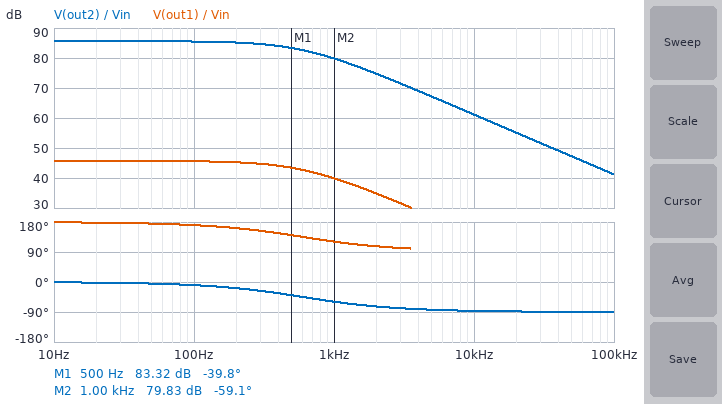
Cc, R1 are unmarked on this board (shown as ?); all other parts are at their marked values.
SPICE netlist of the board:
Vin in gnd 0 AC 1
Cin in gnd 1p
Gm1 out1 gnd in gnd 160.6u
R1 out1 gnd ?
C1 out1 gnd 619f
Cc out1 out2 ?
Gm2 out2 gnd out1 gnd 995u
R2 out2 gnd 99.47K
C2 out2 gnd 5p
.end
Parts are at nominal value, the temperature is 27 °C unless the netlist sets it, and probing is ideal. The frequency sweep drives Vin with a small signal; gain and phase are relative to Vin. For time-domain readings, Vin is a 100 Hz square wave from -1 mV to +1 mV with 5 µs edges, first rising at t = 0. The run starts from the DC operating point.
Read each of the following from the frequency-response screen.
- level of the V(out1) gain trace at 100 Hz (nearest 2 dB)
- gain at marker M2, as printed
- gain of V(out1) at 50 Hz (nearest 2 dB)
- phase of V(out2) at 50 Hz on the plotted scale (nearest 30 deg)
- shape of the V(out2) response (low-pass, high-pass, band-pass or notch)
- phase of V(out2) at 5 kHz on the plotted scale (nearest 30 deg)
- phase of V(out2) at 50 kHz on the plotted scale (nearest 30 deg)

46 dB
79.83 dB
46 dB
0 deg
low-pass
-90 deg
-90 deg
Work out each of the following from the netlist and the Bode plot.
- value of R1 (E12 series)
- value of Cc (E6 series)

1.2 MΩ
2.2 pF
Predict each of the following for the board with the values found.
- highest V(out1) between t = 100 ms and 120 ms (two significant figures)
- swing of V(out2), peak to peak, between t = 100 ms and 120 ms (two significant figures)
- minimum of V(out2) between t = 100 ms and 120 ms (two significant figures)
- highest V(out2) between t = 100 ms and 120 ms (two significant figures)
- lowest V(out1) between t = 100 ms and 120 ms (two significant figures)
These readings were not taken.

190 mV
38 V
-19 V
19 V
-190 mV
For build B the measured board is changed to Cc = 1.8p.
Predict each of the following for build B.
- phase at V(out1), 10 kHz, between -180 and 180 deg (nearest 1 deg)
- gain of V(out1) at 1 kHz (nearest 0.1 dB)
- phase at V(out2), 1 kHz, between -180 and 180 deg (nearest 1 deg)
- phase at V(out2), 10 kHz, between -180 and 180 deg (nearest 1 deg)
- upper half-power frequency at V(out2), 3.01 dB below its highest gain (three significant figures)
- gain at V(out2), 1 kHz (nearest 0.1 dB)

97 deg
41.1 dB
-54 deg
-86 deg
732 Hz
81.0 dB
